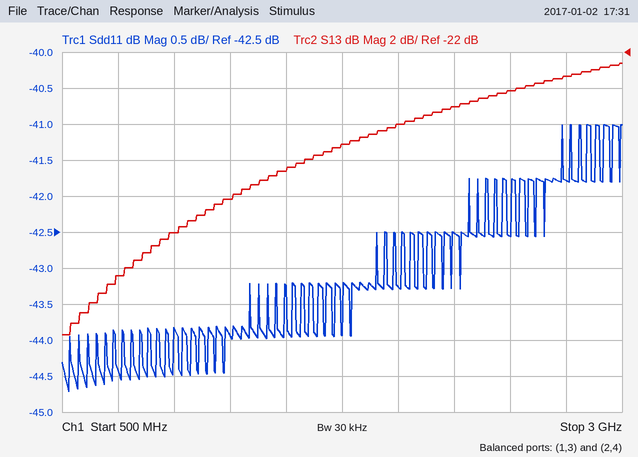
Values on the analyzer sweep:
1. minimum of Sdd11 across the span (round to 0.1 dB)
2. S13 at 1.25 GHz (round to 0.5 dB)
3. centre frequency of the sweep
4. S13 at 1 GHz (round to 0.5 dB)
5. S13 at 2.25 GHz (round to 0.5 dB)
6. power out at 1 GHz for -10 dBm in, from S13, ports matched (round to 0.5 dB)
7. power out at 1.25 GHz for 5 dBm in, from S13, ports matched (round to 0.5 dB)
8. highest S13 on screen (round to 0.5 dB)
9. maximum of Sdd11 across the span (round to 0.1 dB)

-44.7 dB
-30.0 dB
1.75 GHz
-32.0 dB
-25.0 dB
-42.0 dBm
-25.0 dBm
-22.5 dB
-41.0 dB
